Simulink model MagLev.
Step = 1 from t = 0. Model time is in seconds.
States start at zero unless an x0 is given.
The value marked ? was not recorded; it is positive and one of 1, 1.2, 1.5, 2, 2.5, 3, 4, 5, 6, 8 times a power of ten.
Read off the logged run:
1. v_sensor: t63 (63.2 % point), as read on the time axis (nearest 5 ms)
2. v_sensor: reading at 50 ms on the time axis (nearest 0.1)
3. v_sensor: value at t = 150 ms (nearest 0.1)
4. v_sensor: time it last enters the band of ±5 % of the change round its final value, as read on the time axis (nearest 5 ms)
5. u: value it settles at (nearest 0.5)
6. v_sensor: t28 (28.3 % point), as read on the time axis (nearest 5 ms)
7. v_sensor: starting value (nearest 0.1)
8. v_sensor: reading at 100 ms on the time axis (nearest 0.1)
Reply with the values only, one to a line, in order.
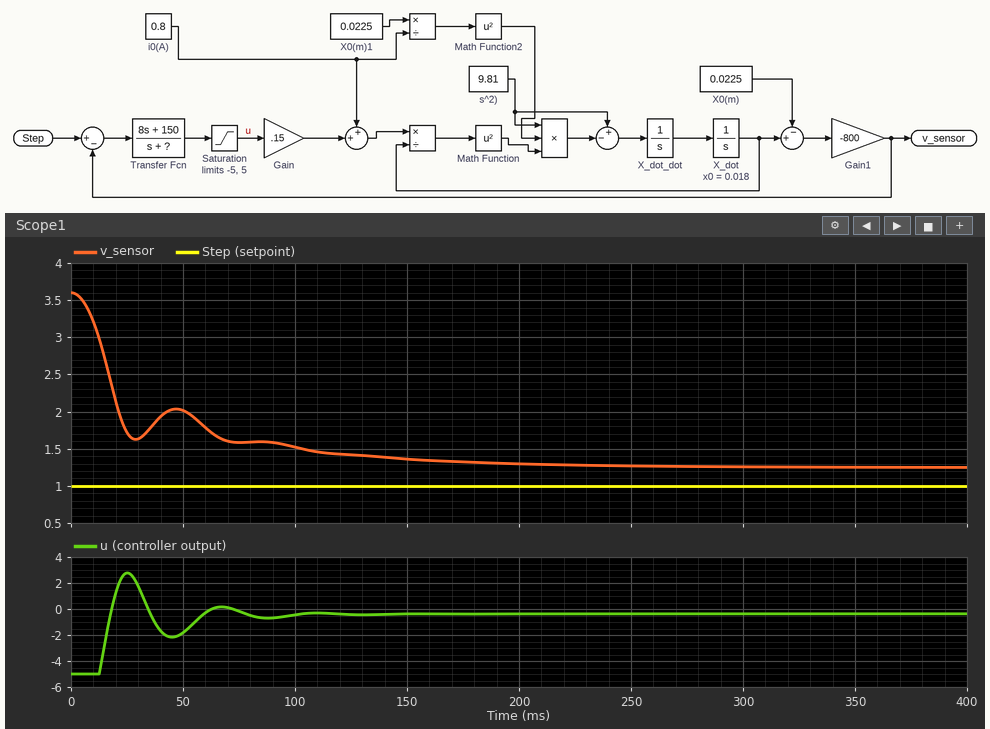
20 ms
2.0
1.4
150 ms
-0.5
15 ms
3.6
1.5
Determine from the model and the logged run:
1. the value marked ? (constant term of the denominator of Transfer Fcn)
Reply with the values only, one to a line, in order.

100
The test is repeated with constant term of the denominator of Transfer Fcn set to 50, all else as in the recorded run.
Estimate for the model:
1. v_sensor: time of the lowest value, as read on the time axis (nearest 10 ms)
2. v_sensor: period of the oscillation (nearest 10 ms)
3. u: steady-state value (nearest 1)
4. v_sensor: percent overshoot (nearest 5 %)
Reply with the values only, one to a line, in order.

30 ms
50 ms
0
10 %
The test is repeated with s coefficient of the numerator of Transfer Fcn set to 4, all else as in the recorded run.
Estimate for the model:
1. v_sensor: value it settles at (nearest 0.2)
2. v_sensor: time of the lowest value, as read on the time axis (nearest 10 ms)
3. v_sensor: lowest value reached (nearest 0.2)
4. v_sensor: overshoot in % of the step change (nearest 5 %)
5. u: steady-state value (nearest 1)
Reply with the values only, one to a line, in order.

1.2
40 ms
0.8
20 %
0
